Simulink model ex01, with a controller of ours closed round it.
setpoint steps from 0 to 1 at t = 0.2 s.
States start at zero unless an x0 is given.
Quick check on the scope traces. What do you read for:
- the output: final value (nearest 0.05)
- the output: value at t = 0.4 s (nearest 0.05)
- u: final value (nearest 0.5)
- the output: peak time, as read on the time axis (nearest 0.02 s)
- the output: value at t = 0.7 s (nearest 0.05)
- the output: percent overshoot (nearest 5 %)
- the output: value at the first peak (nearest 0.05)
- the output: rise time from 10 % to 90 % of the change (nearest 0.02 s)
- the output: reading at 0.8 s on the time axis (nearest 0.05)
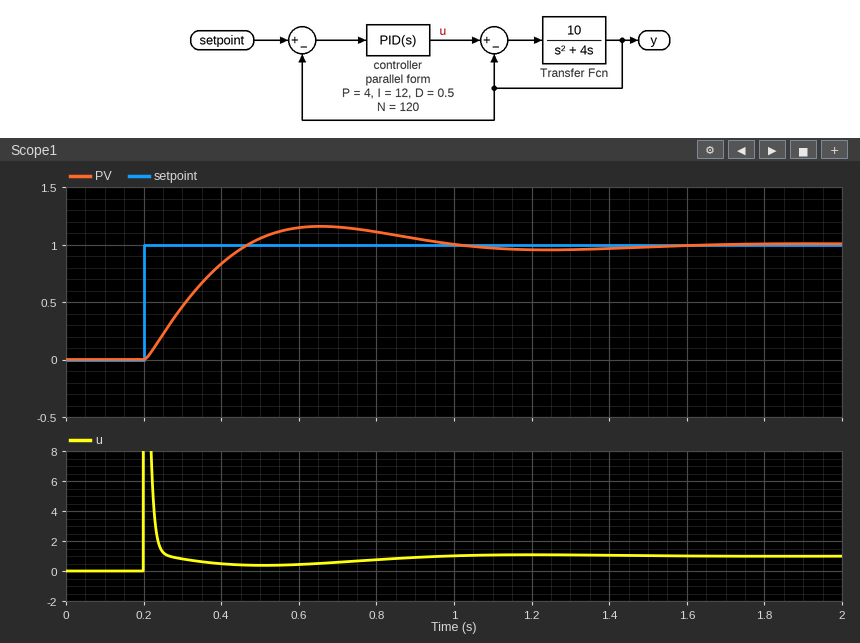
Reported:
1.00
0.85
1.0
0.66 s
1.15
15 %
1.15
0.20 s
1.10
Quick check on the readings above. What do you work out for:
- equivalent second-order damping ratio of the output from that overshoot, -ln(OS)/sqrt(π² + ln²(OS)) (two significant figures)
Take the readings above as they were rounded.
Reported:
0.52
